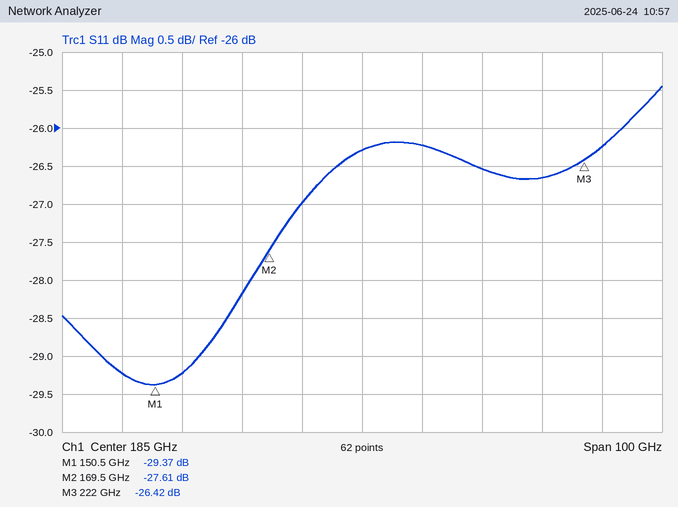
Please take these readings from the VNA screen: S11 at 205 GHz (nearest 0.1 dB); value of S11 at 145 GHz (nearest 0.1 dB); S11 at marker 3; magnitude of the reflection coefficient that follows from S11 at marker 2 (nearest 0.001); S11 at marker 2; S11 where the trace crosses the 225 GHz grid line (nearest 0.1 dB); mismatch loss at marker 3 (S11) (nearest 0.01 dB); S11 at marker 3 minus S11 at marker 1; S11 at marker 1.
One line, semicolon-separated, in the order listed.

-26.5 dB; -29.2 dB; -26.42 dB; 0.042; -27.61 dB; -26.2 dB; 0.01 dB; 2.95 dB; -29.37 dB
